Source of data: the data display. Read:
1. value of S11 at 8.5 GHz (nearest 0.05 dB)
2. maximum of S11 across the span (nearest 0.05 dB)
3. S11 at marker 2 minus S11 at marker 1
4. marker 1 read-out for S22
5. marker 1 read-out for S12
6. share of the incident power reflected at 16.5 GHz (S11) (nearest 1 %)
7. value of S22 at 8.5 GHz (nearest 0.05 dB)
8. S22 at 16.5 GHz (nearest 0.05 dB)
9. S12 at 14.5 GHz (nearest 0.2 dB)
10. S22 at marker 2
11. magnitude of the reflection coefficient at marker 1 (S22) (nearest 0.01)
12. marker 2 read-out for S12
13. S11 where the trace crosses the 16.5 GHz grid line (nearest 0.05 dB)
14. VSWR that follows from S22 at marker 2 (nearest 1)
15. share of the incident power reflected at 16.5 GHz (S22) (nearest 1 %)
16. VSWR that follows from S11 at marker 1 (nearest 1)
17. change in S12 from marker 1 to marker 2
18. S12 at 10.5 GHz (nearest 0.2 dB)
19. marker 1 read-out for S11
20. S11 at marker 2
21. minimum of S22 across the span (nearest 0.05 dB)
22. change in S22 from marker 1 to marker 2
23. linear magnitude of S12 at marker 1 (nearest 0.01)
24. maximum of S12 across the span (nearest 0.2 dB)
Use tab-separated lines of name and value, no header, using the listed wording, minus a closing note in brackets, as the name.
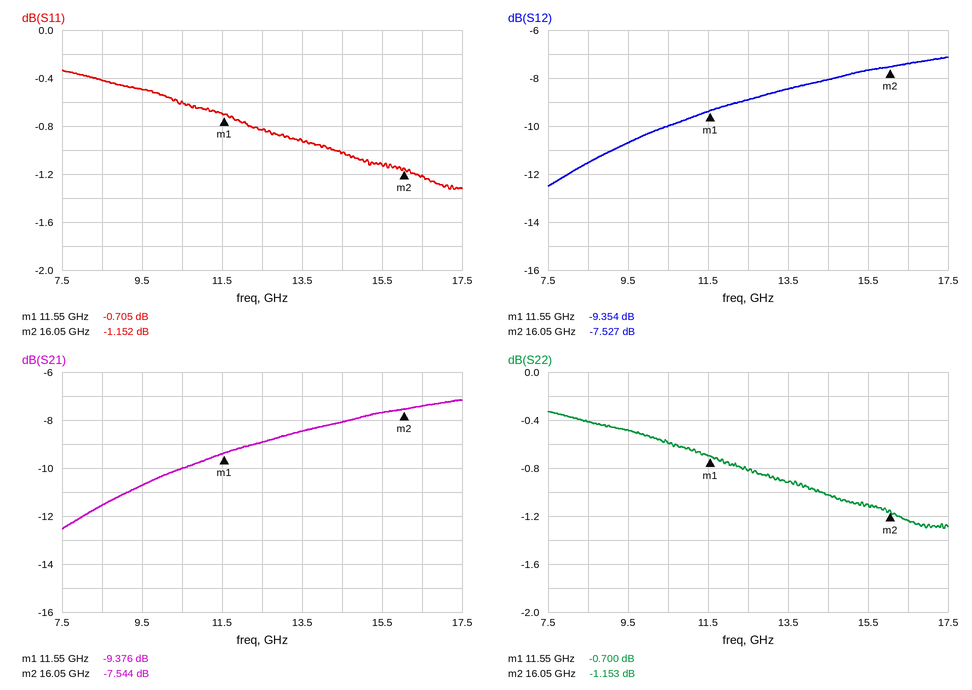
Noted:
value of S11 at 8.5 GHz	-0.40 dB
maximum of S11 across the span	-0.35 dB
S11 at marker 2 minus S11 at marker 1	-0.447 dB
marker 1 read-out for S22	-0.700 dB
marker 1 read-out for S12	-9.354 dB
share of the incident power reflected at 16.5 GHz (S11)	76 %
value of S22 at 8.5 GHz	-0.40 dB
S22 at 16.5 GHz	-1.25 dB
S12 at 14.5 GHz	-8.0 dB
S22 at marker 2	-1.153 dB
magnitude of the reflection coefficient at marker 1 (S22)	0.92
marker 2 read-out for S12	-7.527 dB
S11 where the trace crosses the 16.5 GHz grid line	-1.20 dB
VSWR that follows from S22 at marker 2	15
share of the incident power reflected at 16.5 GHz (S22)	75 %
VSWR that follows from S11 at marker 1	25
change in S12 from marker 1 to marker 2	1.827 dB
S12 at 10.5 GHz	-10.0 dB
marker 1 read-out for S11	-0.705 dB
S11 at marker 2	-1.152 dB
minimum of S22 across the span	-1.30 dB
change in S22 from marker 1 to marker 2	-0.453 dB
linear magnitude of S12 at marker 1	0.34
maximum of S12 across the span	-7.2 dB
